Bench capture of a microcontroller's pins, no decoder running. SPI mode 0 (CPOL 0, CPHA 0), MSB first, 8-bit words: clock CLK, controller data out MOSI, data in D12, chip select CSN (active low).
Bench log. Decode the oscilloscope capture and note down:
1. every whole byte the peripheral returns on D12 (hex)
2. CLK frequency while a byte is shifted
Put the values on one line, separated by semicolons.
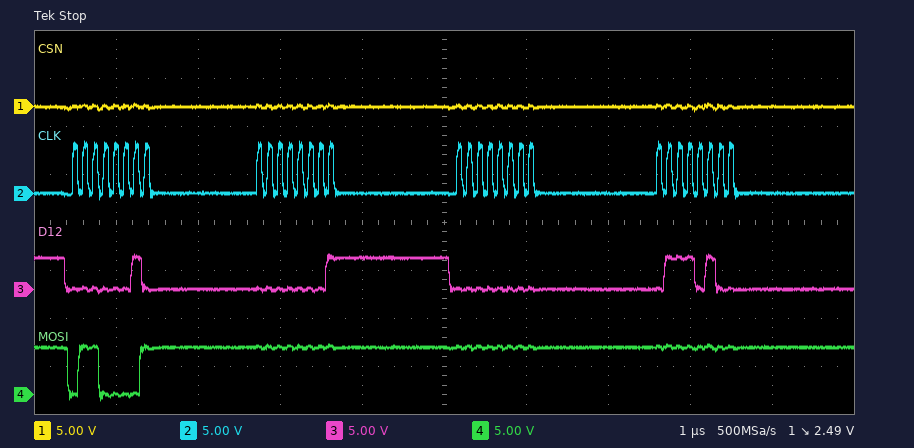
02 01 00 74; 8 MHz
